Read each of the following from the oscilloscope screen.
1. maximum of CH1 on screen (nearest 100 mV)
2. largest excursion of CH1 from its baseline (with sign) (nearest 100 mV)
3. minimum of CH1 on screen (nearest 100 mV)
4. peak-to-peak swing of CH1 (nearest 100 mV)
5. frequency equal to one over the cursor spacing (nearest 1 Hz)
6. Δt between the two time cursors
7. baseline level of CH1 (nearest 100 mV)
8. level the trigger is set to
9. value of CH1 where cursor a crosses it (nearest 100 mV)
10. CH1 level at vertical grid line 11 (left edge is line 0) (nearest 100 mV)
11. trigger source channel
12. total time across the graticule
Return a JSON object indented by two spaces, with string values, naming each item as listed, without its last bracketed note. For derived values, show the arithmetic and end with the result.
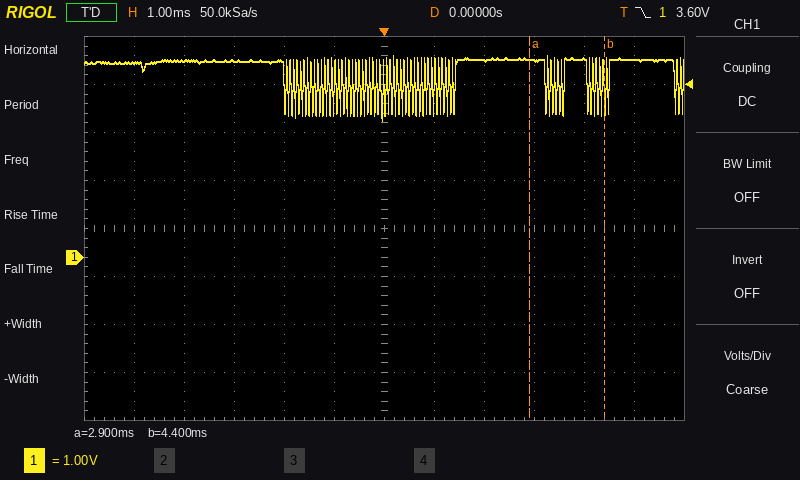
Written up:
{
  "maximum of CH1 on screen": "4.2 V",
  "largest excursion of CH1 from its baseline (with sign)": "2.8 V − (4.1 V) = -1.3 V",
  "minimum of CH1 on screen": "2.8 V",
  "peak-to-peak swing of CH1": "4.2 V − (2.8 V) = 1.4 V",
  "frequency equal to one over the cursor spacing": "1 / 1.5 ms ≈ 667 Hz",
  "Δt between the two time cursors": "4.4 ms − (2.9 ms) = 1.5 ms",
  "baseline level of CH1": "4.1 V",
  "level the trigger is set to": "3.60 V",
  "value of CH1 where cursor a crosses it": "4.1 V",
  "CH1 level at vertical grid line 11 (left edge is line 0)": "4.1 V",
  "trigger source channel": "CH1",
  "total time across the graticule": "12 ms"
}
